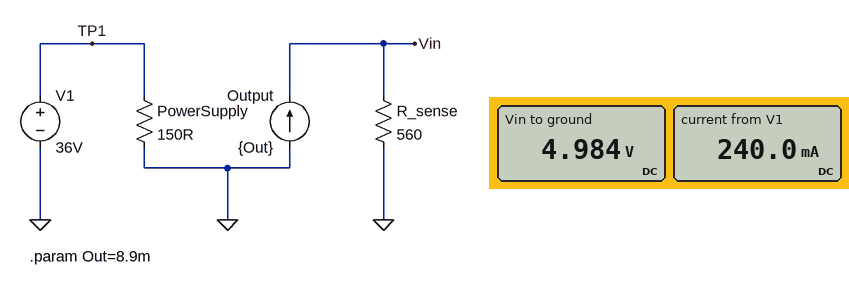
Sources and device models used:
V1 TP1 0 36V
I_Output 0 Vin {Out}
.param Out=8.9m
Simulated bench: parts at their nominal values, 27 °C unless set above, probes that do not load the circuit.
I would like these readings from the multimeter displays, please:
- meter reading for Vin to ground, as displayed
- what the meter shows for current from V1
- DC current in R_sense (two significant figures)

4.984 V
240.0 mA
8.9 mA
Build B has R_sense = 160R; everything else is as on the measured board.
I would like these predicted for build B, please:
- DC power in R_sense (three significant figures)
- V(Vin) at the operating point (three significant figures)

12.7 mW
1.42 V
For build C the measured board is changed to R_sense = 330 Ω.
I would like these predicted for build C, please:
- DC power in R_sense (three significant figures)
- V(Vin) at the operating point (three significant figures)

26.1 mW
2.94 V
